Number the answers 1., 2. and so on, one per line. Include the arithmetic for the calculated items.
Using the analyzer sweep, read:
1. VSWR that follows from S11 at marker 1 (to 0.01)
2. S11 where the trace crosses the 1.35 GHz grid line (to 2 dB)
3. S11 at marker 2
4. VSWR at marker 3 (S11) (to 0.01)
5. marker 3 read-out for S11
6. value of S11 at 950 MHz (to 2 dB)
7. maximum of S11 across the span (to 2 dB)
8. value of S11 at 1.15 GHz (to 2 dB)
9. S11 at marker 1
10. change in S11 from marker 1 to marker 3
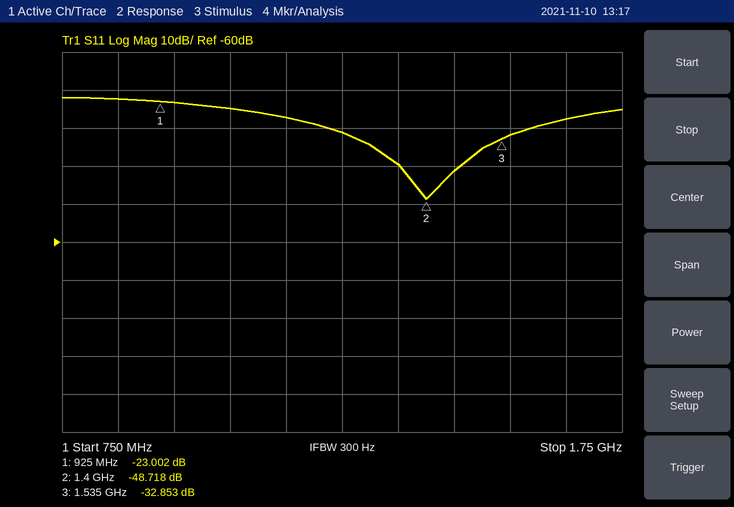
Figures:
1. (1 + 0.0708)/(1 − 0.0708) ≈ 1.15
2. -40 dB
3. -48.718 dB
4. (1 + 0.0228)/(1 − 0.0228) ≈ 1.05
5. -32.853 dB
6. -24 dB
7. -22 dB
8. -28 dB
9. -23.002 dB
10. -32.853 − (-23.002) = -9.851 dB
